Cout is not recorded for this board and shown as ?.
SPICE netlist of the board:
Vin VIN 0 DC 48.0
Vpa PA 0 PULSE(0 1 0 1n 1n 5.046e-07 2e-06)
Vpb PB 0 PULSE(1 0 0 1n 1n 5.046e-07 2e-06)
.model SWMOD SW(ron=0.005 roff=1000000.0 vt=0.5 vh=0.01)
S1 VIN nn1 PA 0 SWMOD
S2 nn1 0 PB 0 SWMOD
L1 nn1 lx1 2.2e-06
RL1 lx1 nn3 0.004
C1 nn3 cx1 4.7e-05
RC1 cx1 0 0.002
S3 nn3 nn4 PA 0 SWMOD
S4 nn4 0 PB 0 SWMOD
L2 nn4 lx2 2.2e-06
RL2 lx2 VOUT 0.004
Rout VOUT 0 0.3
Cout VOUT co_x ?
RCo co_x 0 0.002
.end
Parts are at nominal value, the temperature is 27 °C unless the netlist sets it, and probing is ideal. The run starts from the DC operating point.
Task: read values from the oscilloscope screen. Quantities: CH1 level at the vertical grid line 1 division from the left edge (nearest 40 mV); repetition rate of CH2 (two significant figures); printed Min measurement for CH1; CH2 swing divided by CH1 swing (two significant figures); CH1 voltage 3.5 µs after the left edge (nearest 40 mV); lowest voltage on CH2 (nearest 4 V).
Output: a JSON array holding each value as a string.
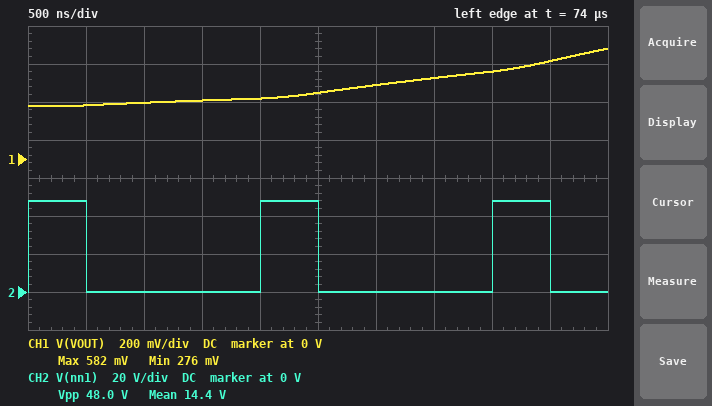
["280 mV", "500 kHz", "276 mV", "160", "440 mV", "0 V"]
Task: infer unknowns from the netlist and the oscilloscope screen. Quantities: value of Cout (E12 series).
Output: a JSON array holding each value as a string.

["33 µF"]
